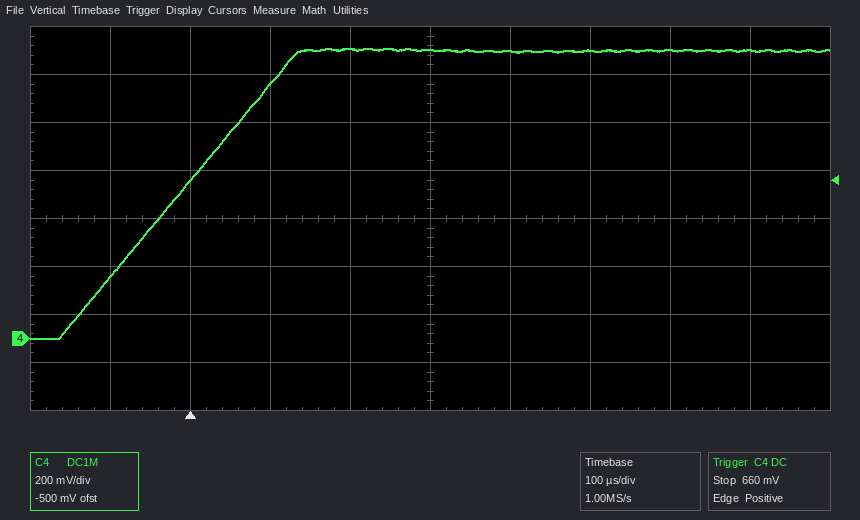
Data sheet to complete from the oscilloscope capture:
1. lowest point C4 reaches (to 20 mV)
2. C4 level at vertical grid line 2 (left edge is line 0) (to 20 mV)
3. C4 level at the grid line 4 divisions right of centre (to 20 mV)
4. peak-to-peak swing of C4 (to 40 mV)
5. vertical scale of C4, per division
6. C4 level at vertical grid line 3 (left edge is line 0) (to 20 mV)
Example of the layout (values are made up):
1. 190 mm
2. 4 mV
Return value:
1. 0 mV
2. 660 mV
3. 1.20 V
4. 1.20 V
5. 200 mV
6. 1.06 V
